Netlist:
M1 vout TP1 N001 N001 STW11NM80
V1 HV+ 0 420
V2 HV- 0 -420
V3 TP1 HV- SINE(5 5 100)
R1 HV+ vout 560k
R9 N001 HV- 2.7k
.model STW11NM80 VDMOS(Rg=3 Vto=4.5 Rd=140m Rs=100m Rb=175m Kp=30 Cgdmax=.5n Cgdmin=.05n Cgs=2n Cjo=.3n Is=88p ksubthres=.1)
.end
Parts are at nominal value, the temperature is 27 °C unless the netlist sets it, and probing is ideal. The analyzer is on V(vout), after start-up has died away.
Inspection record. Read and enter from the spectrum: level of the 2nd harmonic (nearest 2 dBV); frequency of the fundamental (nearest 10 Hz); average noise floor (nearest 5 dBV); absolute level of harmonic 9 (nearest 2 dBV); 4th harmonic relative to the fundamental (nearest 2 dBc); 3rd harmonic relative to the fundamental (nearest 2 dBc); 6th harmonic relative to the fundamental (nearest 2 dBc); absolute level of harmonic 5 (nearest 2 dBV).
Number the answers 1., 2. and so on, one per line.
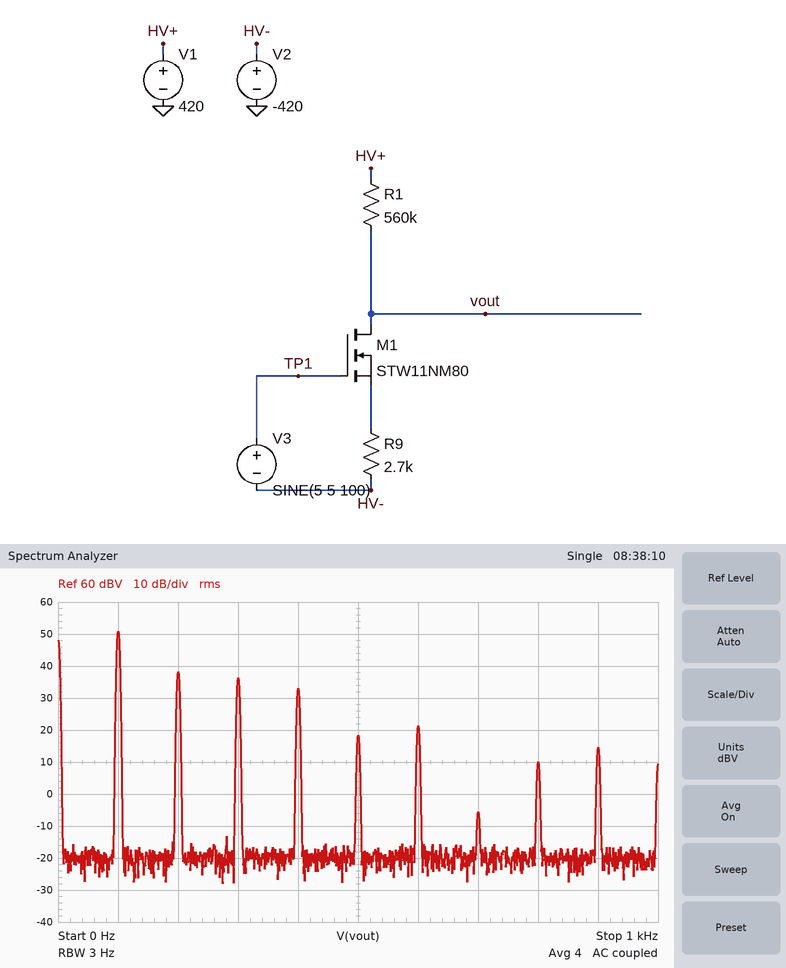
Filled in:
1. 38 dBV
2. 100 Hz
3. -20 dBV
4. 14 dBV
5. -18 dBc
6. -14 dBc
7. -30 dBc
8. 18 dBV
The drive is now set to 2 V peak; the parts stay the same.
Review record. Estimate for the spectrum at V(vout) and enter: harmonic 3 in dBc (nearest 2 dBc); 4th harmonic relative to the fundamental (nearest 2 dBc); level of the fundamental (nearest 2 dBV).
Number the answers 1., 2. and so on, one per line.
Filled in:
1. -22 dBc
2. -50 dBc
3. 46 dBV
